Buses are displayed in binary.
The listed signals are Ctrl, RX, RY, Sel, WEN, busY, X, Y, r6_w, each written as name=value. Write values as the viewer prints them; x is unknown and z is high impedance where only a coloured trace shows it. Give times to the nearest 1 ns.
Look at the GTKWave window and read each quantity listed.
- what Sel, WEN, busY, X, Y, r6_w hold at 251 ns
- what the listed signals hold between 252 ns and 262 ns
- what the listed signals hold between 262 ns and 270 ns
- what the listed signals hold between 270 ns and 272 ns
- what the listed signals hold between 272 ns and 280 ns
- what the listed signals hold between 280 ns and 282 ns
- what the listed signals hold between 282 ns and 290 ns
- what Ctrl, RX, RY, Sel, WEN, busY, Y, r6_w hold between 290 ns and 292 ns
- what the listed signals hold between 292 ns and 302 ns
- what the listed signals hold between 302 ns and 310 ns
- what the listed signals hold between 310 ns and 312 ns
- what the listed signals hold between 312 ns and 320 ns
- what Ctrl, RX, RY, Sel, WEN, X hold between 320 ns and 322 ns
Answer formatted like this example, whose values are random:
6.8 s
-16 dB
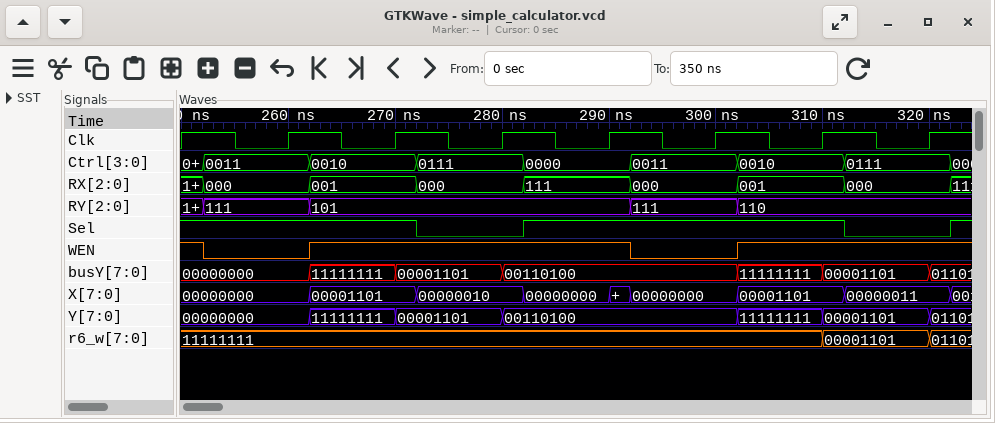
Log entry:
Sel=1, WEN=1, busY=00000000, X=00000000, Y=00000000, r6_w=11111111
Ctrl=0011, RX=000, RY=111, Sel=1, WEN=0, busY=00000000, X=00000000, Y=00000000, r6_w=11111111
Ctrl=0010, RX=001, RY=101, Sel=1, WEN=1, busY=11111111, X=00001101, Y=11111111, r6_w=11111111
Ctrl=0010, RX=001, RY=101, Sel=1, WEN=1, busY=00001101, X=00001101, Y=00001101, r6_w=11111111
Ctrl=0111, RX=000, RY=101, Sel=0, WEN=1, busY=00001101, X=00000010, Y=00001101, r6_w=11111111
Ctrl=0111, RX=000, RY=101, Sel=0, WEN=1, busY=00110100, X=00000010, Y=00110100, r6_w=11111111
Ctrl=0000, RX=111, RY=101, Sel=1, WEN=1, busY=00110100, X=00000000, Y=00110100, r6_w=11111111
Ctrl=0000, RX=111, RY=101, Sel=1, WEN=1, busY=00110100, Y=00110100, r6_w=11111111
Ctrl=0011, RX=000, RY=111, Sel=1, WEN=0, busY=00110100, X=00000000, Y=00110100, r6_w=11111111
Ctrl=0010, RX=001, RY=110, Sel=1, WEN=1, busY=11111111, X=00001101, Y=11111111, r6_w=11111111
Ctrl=0010, RX=001, RY=110, Sel=1, WEN=1, busY=00001101, X=00001101, Y=00001101, r6_w=00001101
Ctrl=0111, RX=000, RY=110, Sel=0, WEN=1, busY=00001101, X=00000011, Y=00001101, r6_w=00001101
Ctrl=0111, RX=000, RY=110, Sel=0, WEN=1, X=00000011
